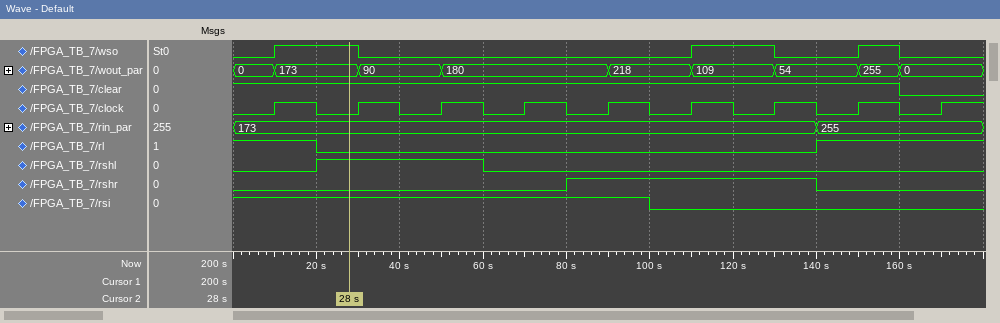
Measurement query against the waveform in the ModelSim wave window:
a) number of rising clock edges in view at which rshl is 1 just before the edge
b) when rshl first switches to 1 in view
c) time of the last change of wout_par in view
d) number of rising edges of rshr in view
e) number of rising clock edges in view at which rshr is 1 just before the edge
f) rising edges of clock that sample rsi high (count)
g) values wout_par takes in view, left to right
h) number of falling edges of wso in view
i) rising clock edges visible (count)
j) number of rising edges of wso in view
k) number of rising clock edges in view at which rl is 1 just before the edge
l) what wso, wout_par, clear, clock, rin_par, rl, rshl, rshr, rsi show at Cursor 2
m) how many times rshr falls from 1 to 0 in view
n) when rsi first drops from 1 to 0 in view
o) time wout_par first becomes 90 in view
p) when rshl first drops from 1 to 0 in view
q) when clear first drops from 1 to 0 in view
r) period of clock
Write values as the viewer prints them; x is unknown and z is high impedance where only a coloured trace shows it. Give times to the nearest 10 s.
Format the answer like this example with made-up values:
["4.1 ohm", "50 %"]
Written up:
["2", "20 s", "160 s", "1", "3", "5", "0, 173, 90, 180, 218, 109, 54, 255, 0", "3", "9", "3", "3", "wso=1, wout_par=173, clear=1, clock=0, rin_par=173, rl=0, rshl=1, rshr=0, rsi=1", "1", "100 s", "30 s", "60 s", "160 s", "20 s"]
